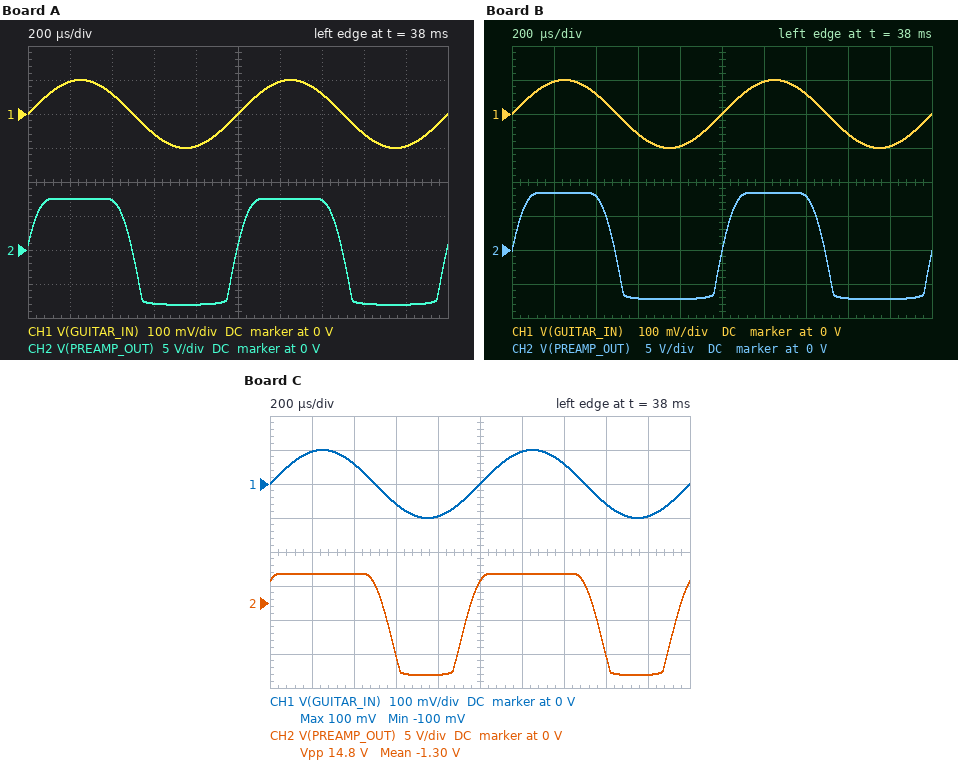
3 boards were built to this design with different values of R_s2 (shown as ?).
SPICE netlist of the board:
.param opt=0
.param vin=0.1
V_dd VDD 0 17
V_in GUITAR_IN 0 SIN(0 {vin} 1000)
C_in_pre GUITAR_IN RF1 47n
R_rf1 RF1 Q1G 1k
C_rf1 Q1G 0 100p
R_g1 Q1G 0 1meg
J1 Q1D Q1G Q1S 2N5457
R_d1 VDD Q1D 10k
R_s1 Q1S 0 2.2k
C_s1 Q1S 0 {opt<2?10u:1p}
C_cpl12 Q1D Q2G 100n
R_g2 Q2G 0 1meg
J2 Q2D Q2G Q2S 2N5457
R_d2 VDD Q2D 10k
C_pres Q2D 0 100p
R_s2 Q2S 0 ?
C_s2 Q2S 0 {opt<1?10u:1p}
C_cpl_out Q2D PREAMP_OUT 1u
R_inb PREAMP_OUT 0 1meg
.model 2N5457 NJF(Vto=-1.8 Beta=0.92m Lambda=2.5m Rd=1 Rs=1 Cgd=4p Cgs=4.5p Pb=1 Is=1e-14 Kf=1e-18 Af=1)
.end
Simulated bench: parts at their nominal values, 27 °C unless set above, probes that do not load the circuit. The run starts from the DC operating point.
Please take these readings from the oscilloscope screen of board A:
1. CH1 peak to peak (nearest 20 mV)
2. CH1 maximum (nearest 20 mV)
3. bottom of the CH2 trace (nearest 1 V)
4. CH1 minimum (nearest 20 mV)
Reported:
200 mV
100 mV
-8 V
-100 mV
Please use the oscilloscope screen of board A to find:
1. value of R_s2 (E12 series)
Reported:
1.2 kΩ
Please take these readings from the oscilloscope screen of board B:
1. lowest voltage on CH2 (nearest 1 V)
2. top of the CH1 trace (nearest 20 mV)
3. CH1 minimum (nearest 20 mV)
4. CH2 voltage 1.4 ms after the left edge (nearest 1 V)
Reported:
-7 V
100 mV
-100 mV
8 V
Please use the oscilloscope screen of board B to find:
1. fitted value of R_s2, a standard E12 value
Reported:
1 kΩ
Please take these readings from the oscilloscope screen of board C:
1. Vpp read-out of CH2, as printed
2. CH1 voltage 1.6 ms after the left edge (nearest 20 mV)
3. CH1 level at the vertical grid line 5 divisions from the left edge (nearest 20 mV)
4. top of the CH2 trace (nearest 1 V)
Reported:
14.8 V
-60 mV
0 V
4 V
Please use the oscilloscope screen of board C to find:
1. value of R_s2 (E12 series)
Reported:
2.7 kΩ
